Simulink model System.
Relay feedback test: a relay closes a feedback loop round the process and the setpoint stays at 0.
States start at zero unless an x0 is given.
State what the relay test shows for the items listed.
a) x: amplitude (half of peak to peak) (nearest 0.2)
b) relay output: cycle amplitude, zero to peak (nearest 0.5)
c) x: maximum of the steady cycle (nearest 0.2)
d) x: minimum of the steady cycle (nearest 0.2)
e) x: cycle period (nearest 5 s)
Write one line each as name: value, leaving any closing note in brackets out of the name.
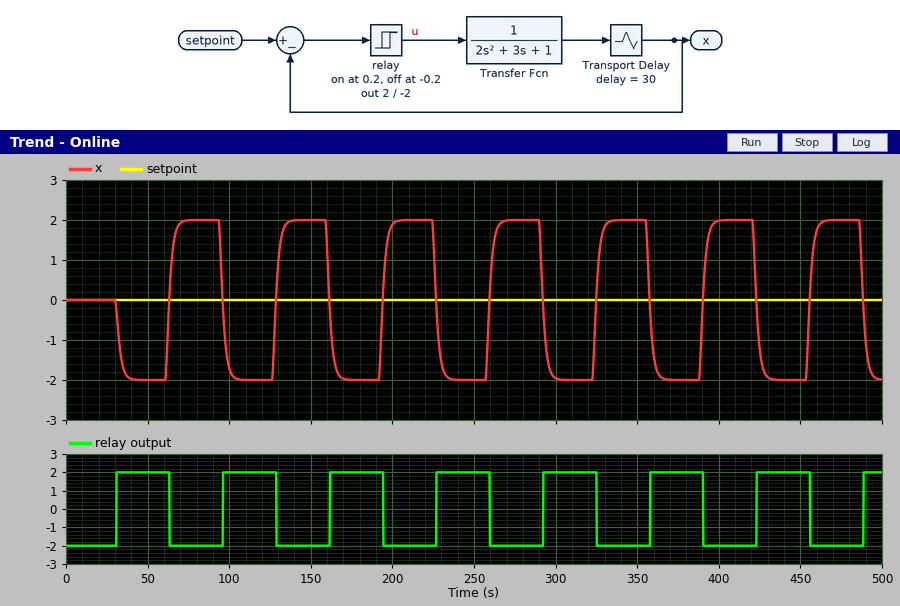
x: amplitude (half of peak to peak): 2.0
relay output: cycle amplitude, zero to peak: 2.0
x: maximum of the steady cycle: 2.0
x: minimum of the steady cycle: -2.0
x: cycle period: 65 s
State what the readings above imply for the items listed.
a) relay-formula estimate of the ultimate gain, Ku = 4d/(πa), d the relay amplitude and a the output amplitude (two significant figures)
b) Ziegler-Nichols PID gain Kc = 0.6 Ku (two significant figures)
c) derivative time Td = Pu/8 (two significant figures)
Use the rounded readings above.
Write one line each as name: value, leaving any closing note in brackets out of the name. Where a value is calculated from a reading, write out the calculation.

relay-formula estimate of the ultimate gain, Ku = 4d/(πa), d the relay amplitude and a the output amplitude: 4 × 2 / (π × 2) = 1.3
Ziegler-Nichols PID gain Kc = 0.6 Ku: 0.6 × 1.3 = 0.78
derivative time Td = Pu/8: 65 / 8 = 8.1 s
